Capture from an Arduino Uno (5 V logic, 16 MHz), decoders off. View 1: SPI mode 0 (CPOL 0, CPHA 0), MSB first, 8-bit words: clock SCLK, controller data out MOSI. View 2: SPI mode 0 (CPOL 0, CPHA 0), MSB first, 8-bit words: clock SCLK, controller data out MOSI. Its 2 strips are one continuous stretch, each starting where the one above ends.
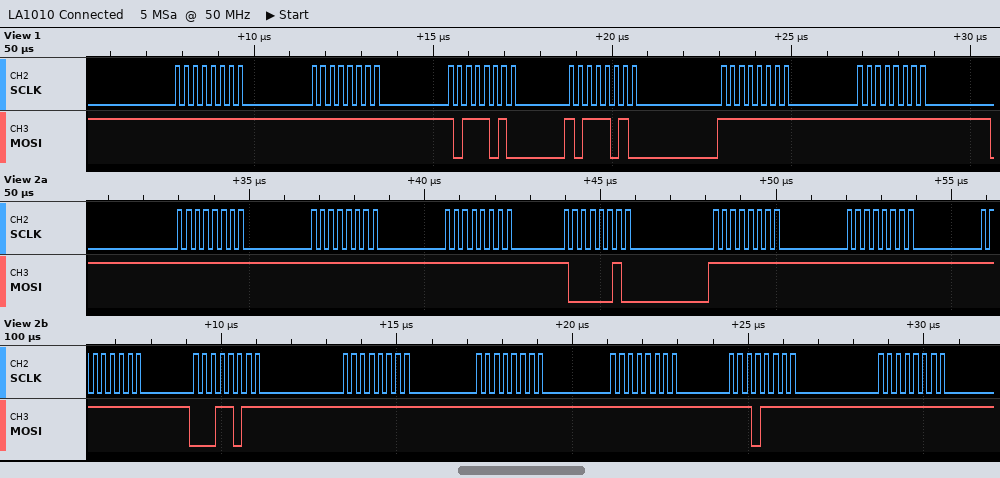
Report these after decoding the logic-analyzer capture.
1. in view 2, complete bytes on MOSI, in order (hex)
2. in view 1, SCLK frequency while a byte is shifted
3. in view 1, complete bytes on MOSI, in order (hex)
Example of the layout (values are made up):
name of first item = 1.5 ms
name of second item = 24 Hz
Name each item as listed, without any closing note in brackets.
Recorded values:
in view 2, complete bytes on MOSI, in order = FF FF FF 82 FF FF FF 1B FF FF FF EF FF
in view 1, SCLK frequency while a byte is shifted = 4 MHz
in view 1, complete bytes on MOSI, in order = 0xFF 0xFF 0xBA 0xBA 0xFF 0xFF
